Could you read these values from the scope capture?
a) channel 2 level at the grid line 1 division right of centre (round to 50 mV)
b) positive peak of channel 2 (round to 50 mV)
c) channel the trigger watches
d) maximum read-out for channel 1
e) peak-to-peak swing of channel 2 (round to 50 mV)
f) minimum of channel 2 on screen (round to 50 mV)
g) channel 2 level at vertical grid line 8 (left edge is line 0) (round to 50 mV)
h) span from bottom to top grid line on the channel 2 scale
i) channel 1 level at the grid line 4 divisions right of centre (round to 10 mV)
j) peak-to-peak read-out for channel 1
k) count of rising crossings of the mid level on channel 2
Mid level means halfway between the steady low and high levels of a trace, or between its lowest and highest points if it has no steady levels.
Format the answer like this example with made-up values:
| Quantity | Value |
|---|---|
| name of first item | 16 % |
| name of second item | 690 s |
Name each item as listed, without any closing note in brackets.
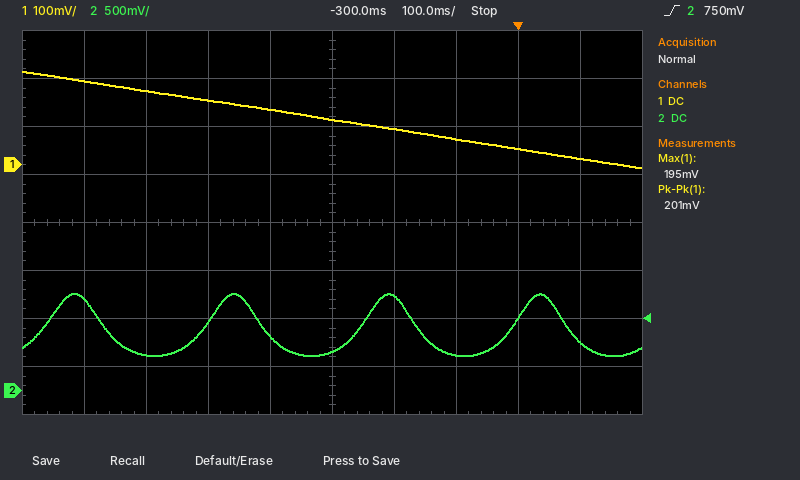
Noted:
| Quantity | Value |
|---|---|
| channel 2 level at the grid line 1 division right of centre | 1.00 V |
| positive peak of channel 2 | 1.00 V |
| channel the trigger watches | channel 2 |
| maximum read-out for channel 1 | 195 mV |
| peak-to-peak swing of channel 2 | 650 mV |
| minimum of channel 2 on screen | 350 mV |
| channel 2 level at vertical grid line 8 (left edge is line 0) | 750 mV |
| span from bottom to top grid line on the channel 2 scale | 4 V |
| channel 1 level at the grid line 4 divisions right of centre | 10 mV |
| peak-to-peak read-out for channel 1 | 201 mV |
| count of rising crossings of the mid level on channel 2 | 4 |
